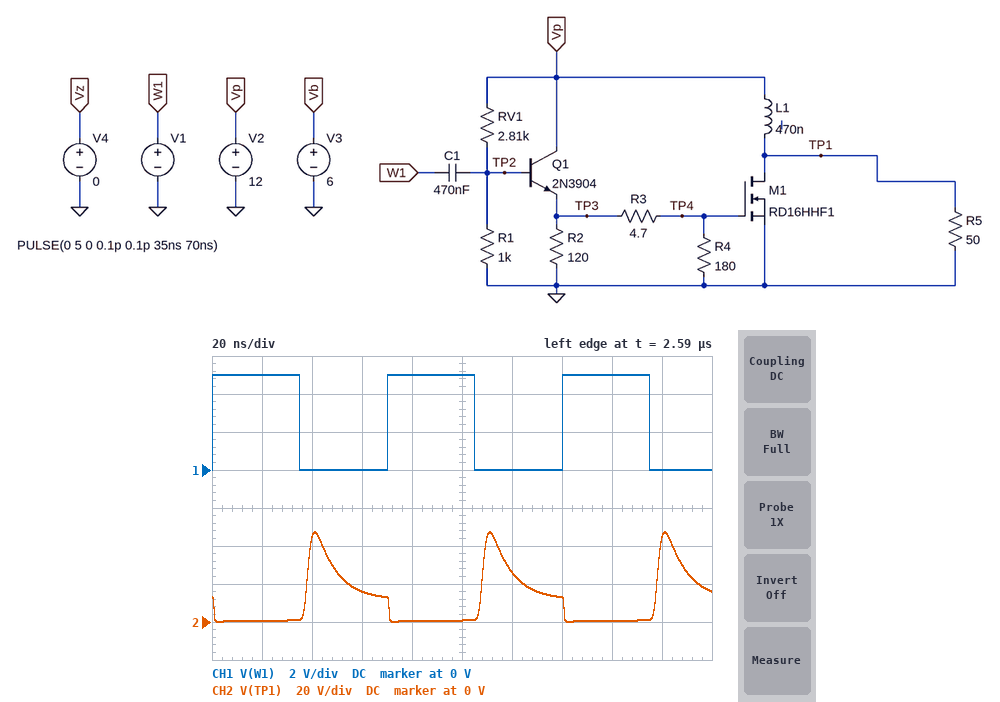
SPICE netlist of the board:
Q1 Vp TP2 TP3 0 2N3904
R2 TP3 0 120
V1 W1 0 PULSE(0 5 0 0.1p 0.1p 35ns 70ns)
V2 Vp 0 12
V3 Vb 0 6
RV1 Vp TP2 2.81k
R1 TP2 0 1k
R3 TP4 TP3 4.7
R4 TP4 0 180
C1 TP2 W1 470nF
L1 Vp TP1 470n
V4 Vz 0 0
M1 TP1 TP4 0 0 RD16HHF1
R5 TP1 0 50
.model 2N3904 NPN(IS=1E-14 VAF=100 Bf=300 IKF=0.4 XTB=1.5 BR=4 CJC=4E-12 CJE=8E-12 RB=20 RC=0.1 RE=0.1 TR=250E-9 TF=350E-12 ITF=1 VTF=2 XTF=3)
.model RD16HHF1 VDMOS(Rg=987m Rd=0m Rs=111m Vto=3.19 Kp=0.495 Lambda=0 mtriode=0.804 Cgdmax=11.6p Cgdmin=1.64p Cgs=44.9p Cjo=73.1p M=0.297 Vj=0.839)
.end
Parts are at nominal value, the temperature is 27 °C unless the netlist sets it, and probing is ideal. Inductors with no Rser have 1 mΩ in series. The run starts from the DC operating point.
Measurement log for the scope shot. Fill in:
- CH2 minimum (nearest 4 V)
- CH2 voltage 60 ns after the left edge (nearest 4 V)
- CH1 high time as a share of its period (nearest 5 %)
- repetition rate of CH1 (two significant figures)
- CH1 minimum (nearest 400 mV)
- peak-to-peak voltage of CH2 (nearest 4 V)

0 V
16 V
50 %
14 MHz
0 V
48 V
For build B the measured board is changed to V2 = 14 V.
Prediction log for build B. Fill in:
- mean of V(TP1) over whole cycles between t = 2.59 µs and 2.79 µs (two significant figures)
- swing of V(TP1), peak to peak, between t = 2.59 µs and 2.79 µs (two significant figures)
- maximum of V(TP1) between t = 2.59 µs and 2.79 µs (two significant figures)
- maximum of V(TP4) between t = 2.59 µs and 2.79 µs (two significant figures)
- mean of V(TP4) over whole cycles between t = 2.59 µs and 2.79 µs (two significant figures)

14 V
55 V
56 V
8.3 V
5.3 V
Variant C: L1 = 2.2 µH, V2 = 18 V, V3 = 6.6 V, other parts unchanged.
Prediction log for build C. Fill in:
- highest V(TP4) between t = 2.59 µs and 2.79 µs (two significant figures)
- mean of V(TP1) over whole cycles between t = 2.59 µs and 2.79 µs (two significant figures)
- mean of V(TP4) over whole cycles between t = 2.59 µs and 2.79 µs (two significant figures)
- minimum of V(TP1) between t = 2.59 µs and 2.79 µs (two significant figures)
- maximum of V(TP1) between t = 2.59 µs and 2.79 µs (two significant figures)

9.4 V
18 V
6.2 V
380 mV
45 V
